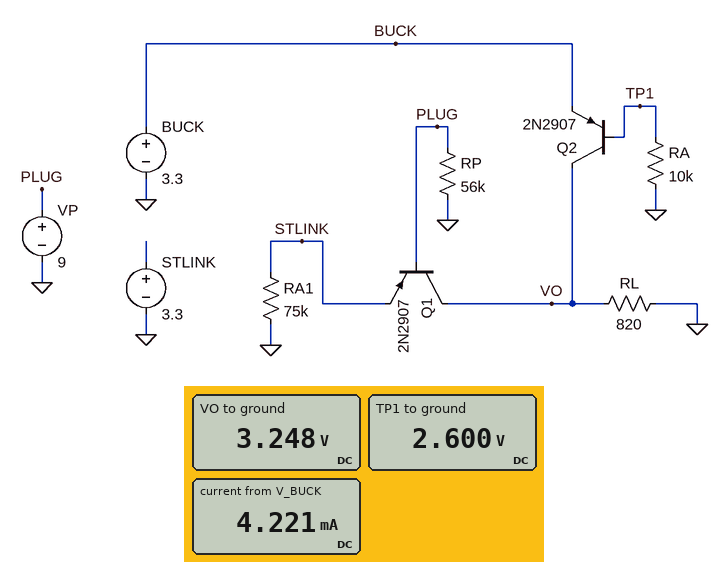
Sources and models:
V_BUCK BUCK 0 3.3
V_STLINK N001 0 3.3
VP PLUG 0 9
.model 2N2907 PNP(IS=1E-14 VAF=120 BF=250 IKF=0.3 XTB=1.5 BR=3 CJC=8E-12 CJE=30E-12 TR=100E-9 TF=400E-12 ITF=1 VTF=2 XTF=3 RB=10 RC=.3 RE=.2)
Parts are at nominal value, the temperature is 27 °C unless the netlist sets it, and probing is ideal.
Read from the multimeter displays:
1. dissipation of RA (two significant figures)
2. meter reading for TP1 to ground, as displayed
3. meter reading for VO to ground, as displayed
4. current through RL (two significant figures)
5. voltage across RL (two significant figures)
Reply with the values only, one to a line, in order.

680 µW
2.600 V
3.248 V
4.0 mA
3.2 V
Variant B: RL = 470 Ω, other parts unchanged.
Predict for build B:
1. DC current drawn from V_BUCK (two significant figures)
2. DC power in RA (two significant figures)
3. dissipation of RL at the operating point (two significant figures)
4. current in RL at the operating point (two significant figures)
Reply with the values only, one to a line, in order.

7.1 mA
670 µW
22 mW
6.9 mA
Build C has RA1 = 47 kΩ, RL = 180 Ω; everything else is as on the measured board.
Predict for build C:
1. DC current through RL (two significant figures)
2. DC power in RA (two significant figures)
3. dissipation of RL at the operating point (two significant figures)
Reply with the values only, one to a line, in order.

18 mA
660 µW
57 mW
